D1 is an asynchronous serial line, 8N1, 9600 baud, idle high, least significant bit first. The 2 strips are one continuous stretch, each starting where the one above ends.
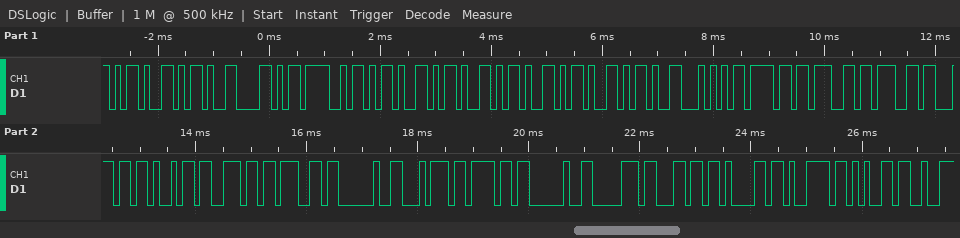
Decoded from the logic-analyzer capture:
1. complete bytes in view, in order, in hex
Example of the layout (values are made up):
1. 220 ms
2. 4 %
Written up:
1. 2D 2D 58 4F 2D 2D 2D 2D 2D 54 6F 67 67 6C 69 6E 67 20 74 6F 20 70 6C 61 79 65
